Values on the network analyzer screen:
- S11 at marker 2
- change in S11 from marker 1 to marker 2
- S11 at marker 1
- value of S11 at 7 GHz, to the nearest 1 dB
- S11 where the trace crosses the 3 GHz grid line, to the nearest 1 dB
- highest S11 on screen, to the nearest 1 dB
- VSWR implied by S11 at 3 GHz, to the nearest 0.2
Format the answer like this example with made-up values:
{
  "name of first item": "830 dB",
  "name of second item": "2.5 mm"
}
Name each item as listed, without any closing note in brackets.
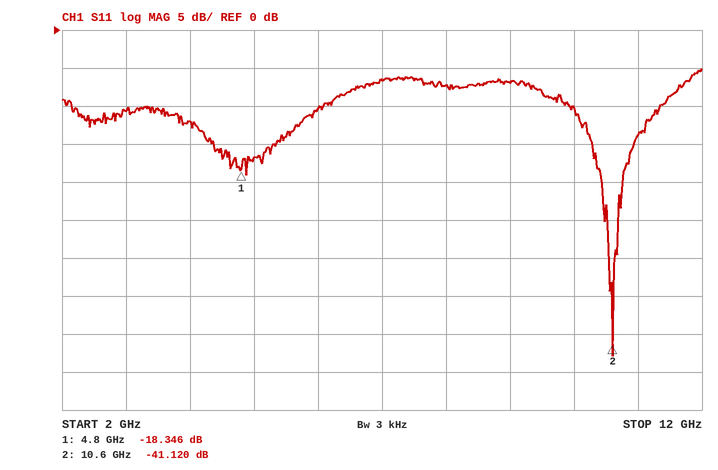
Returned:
{
  "S11 at marker 2": "-41.120 dB",
  "change in S11 from marker 1 to marker 2": "-22.774 dB",
  "S11 at marker 1": "-18.346 dB",
  "value of S11 at 7 GHz, to the nearest 1 dB": "-7 dB",
  "S11 where the trace crosses the 3 GHz grid line, to the nearest 1 dB": "-11 dB",
  "highest S11 on screen, to the nearest 1 dB": "-5 dB",
  "VSWR implied by S11 at 3 GHz, to the nearest 0.2": "1.8"
}
